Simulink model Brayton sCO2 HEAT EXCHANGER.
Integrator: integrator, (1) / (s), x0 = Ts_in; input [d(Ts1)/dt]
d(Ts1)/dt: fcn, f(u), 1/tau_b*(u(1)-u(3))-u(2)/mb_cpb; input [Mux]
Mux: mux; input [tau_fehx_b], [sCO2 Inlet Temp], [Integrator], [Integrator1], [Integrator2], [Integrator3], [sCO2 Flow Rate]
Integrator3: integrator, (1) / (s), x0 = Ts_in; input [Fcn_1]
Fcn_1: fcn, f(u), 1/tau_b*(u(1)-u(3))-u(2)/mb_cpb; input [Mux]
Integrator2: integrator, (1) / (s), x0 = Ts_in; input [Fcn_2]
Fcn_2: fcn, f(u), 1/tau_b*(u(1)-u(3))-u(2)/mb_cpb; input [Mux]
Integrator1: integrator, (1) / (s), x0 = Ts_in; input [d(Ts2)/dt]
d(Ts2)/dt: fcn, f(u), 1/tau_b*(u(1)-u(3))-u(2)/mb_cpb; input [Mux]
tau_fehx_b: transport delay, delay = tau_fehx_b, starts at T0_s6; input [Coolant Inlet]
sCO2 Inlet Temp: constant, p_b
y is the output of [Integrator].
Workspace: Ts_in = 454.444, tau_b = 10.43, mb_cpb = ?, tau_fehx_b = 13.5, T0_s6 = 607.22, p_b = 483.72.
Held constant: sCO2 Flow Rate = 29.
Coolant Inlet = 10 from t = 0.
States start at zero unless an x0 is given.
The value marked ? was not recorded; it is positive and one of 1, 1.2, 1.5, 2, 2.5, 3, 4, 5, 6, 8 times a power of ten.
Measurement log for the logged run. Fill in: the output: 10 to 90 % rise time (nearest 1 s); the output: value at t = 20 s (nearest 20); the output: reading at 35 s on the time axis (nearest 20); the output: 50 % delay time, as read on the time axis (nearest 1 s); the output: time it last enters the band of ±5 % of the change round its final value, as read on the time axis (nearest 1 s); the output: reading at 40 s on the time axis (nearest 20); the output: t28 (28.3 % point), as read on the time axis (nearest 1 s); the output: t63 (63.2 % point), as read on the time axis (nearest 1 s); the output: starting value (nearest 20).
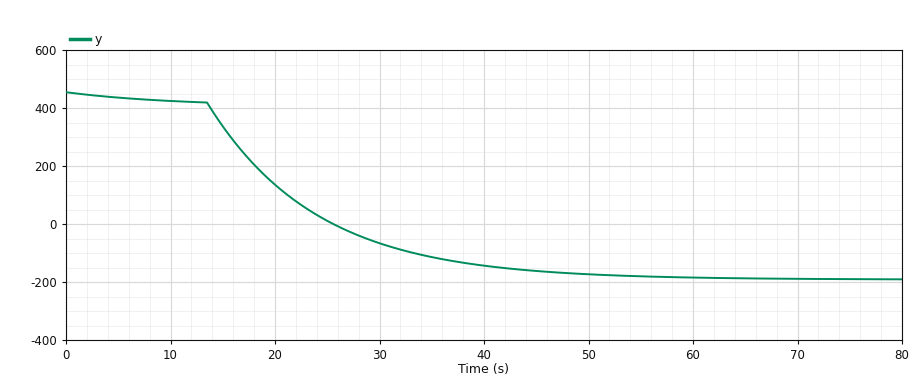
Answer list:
23 s
140
-120
20 s
44 s
-140
16 s
23 s
460
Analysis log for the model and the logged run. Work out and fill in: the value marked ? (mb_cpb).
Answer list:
25
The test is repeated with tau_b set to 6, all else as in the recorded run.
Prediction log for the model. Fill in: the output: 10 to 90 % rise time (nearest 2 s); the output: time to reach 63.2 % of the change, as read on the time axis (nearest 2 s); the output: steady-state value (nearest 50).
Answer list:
14 s
20 s
-100
